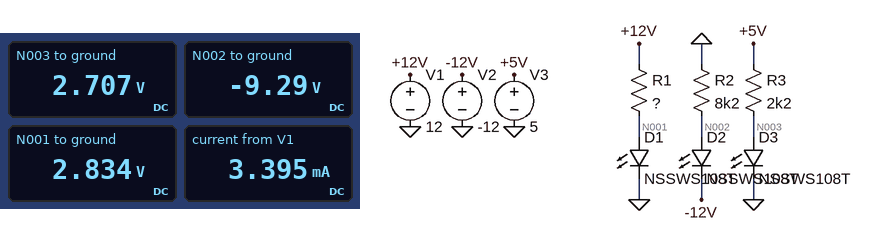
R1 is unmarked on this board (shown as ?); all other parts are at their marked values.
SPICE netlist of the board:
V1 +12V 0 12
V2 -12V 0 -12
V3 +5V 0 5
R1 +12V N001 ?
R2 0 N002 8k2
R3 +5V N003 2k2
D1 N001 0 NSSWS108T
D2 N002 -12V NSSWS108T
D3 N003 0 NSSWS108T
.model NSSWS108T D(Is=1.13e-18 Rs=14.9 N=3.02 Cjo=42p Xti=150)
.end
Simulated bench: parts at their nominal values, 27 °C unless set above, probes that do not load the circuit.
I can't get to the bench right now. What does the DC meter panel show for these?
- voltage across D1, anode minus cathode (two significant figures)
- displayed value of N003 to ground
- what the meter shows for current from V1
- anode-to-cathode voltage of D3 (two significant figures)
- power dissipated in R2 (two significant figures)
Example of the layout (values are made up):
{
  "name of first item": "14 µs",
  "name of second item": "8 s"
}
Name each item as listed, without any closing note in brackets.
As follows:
{
  "voltage across D1, anode minus cathode": "2.8 V",
  "displayed value of N003 to ground": "2.707 V",
  "what the meter shows for current from V1": "3.395 mA",
  "anode-to-cathode voltage of D3": "2.7 V",
  "power dissipated in R2": "11 mW"
}
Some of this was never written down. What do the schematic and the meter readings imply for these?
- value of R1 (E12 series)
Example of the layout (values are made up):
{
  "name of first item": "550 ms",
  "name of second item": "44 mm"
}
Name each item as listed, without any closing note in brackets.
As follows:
{
  "value of R1": "2.7 kΩ"
}
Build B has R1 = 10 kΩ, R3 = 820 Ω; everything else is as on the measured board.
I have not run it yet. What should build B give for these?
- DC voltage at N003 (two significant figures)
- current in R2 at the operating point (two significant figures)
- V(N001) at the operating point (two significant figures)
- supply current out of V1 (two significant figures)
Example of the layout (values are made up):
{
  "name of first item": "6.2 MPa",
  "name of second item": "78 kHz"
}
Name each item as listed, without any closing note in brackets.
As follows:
{
  "DC voltage at N003": "2.8 V",
  "current in R2 at the operating point": "1.1 mA",
  "V(N001) at the operating point": "2.7 V",
  "supply current out of V1": "930 µA"
}
